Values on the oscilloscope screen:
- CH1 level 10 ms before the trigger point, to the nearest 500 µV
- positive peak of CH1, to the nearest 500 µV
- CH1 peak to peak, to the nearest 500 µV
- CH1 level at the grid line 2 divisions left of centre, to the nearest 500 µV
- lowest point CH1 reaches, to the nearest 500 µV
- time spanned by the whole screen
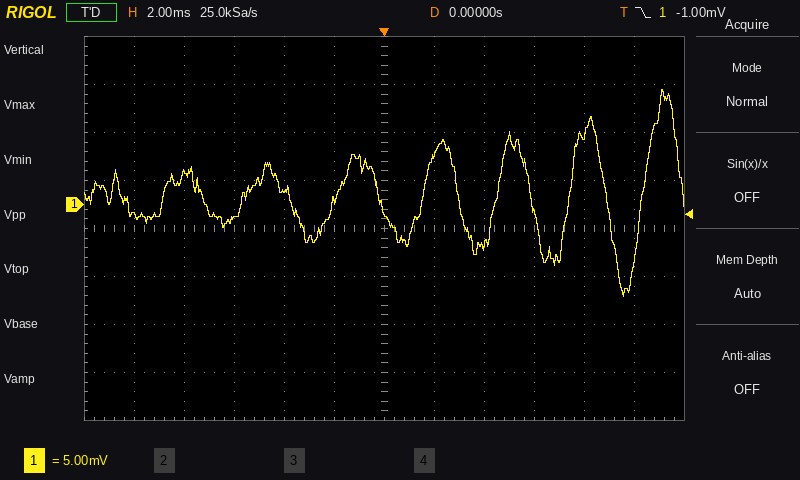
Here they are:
-1.0 mV
12.0 mV
21.5 mV
1.5 mV
-9.5 mV
24 ms
